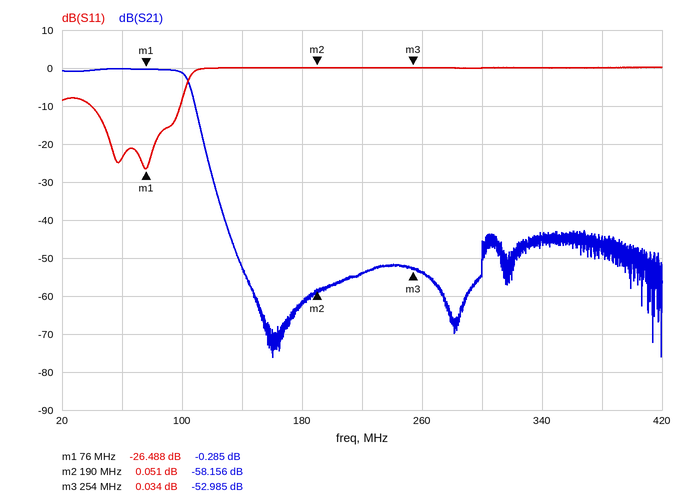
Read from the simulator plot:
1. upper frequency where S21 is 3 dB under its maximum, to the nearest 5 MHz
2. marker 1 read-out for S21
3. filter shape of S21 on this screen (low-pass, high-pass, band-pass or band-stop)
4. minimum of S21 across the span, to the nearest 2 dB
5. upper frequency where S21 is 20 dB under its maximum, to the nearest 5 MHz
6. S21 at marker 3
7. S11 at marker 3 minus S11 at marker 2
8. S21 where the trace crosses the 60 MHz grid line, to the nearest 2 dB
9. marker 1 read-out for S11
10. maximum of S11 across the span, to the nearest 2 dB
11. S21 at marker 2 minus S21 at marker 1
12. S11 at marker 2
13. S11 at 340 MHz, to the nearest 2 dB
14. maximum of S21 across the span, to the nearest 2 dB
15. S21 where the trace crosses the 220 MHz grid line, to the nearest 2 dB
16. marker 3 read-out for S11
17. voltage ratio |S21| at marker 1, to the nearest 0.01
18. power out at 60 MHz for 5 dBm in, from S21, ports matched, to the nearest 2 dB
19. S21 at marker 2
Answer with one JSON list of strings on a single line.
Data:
["105 MHz", "-0.285 dB", "low-pass", "-76 dB", "115 MHz", "-52.985 dB", "-0.017 dB", "0 dB", "-26.488 dB", "0 dB", "-57.871 dB", "0.051 dB", "0 dB", "0 dB", "-54 dB", "0.034 dB", "0.97", "4 dBm", "-58.156 dB"]
